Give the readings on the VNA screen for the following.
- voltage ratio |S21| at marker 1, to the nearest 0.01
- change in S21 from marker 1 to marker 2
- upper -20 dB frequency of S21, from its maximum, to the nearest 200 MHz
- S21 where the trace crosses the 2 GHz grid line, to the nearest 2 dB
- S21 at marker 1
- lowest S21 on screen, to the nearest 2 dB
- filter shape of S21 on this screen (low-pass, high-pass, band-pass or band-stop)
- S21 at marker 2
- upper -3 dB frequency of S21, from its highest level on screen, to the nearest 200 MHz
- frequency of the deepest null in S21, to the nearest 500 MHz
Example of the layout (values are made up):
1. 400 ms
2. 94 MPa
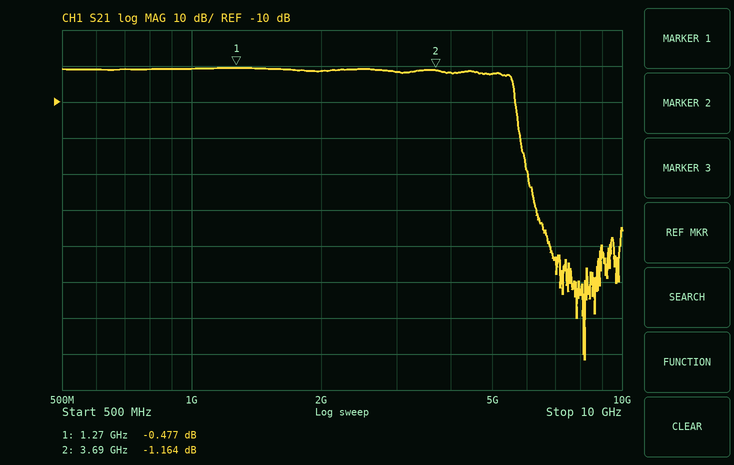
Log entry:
1. 0.95
2. -0.687 dB
3. 5.8 GHz
4. -2 dB
5. -0.477 dB
6. -82 dB
7. low-pass
8. -1.164 dB
9. 5.6 GHz
10. 8.0 GHz
